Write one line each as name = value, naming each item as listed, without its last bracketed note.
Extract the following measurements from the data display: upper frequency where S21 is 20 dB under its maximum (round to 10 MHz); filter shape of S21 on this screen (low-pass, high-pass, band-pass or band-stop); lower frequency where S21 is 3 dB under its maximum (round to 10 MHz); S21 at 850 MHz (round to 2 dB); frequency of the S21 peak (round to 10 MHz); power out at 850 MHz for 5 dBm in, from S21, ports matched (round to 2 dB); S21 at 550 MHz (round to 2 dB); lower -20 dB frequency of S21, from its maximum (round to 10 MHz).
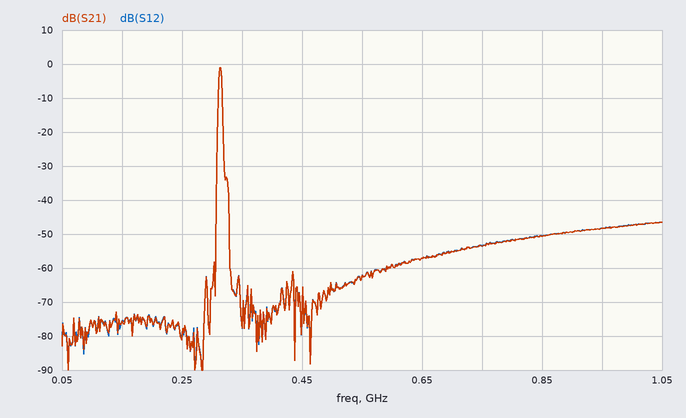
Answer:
upper frequency where S21 is 20 dB under its maximum = 320 MHz
filter shape of S21 on this screen = band-pass
lower frequency where S21 is 3 dB under its maximum = 310 MHz
S21 at 850 MHz = -50 dB
frequency of the S21 peak = 310 MHz
power out at 850 MHz for 5 dBm in, from S21, ports matched = -46 dBm
S21 at 550 MHz = -62 dB
lower -20 dB frequency of S21, from its maximum = 310 MHz
